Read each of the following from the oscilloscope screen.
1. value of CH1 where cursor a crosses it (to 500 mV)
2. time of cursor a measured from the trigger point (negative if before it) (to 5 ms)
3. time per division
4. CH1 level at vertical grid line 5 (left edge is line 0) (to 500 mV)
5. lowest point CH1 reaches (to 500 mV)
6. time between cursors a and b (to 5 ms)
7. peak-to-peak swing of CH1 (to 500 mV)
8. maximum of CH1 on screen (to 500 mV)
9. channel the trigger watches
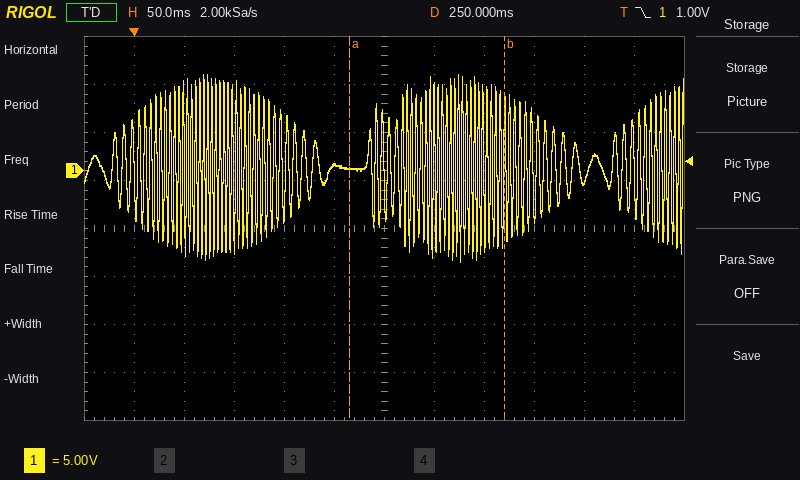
500 mV
+215 ms
50 ms
500 mV
-9.5 V
155 ms
19.5 V
10.0 V
CH1
